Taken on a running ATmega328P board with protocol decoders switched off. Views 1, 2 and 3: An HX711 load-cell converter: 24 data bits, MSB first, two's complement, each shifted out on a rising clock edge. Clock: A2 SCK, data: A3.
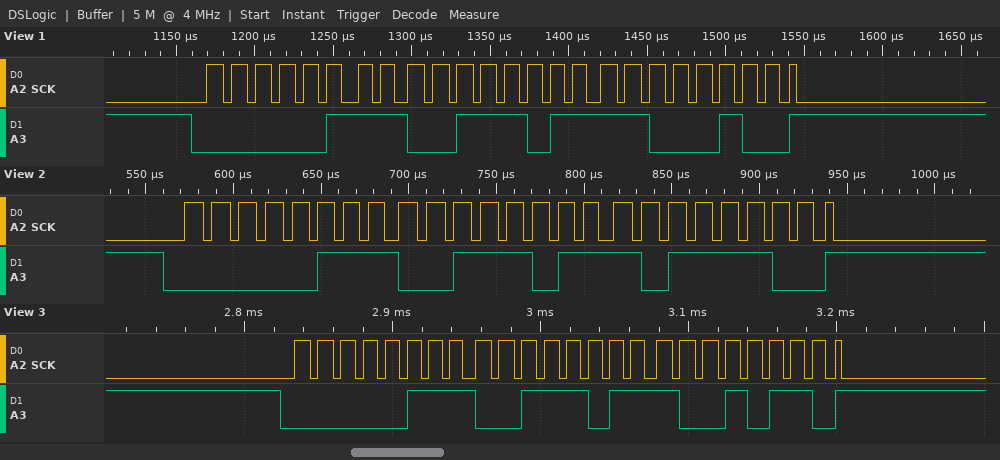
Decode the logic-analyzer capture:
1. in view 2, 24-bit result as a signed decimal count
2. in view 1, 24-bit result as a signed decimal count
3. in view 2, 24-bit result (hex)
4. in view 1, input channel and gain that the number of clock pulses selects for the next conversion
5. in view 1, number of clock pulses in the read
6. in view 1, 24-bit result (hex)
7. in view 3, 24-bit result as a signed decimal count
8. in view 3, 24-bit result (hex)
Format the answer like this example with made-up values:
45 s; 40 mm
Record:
474044; 474052; 0x073BBC; channel A, gain 128; 25; 0x073BC4; 474006; 0x073B96
